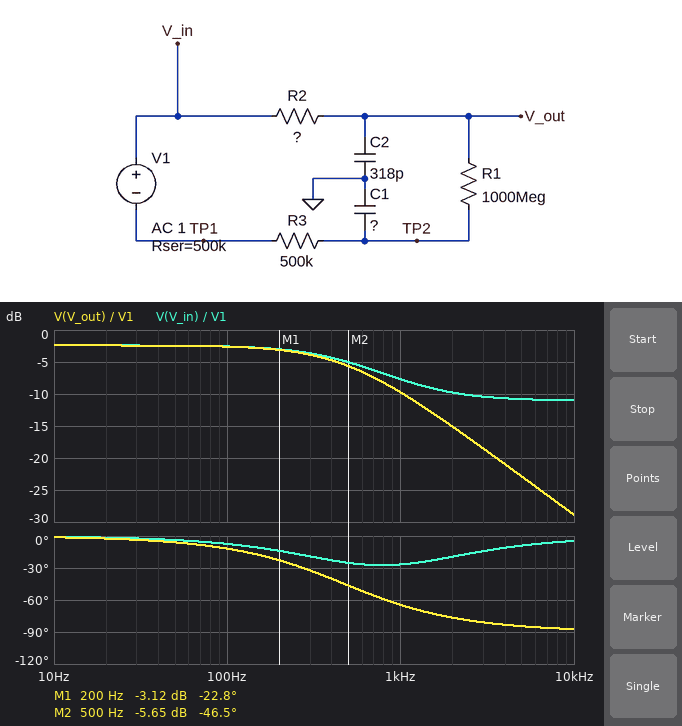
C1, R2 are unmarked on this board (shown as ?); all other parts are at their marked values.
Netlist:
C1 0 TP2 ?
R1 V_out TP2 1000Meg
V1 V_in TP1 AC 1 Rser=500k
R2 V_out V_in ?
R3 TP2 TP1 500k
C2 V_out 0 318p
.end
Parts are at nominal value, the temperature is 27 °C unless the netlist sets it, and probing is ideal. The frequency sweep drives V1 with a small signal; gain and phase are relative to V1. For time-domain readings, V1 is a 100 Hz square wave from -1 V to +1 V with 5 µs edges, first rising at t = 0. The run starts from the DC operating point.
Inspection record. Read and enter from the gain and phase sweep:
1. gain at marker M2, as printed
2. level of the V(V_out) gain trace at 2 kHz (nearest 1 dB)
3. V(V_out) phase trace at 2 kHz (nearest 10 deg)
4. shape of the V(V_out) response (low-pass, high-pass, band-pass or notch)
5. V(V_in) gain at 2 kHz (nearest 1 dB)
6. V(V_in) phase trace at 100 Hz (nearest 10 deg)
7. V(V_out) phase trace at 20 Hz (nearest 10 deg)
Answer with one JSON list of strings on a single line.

["-5.65 dB", "-15 dB", "-80 deg", "low-pass", "-10 dB", "-10 deg", "0 deg"]
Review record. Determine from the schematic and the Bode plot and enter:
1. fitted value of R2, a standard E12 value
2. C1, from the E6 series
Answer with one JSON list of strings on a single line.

["390 kΩ", "1 nF"]
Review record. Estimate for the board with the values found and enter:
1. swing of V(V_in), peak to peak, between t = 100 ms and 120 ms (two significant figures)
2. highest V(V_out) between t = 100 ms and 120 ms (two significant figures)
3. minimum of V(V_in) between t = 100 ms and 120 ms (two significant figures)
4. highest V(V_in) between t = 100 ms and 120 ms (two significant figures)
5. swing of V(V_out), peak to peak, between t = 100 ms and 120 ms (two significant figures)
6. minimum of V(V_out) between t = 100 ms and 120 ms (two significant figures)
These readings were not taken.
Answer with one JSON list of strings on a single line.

["1.5 V", "1.6 V", "57 mV", "1.6 V", "1.5 V", "57 mV"]
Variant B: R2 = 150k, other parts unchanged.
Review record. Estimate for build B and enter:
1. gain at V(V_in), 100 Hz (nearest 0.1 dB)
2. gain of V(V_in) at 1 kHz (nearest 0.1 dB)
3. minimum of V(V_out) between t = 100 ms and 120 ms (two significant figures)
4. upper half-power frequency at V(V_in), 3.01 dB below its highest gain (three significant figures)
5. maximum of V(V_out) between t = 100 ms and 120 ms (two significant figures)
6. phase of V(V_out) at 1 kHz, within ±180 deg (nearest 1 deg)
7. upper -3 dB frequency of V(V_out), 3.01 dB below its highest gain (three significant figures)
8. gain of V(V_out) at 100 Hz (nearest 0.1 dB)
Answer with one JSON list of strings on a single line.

["-2.5 dB", "-8.1 dB", "24 mV", "592 Hz", "1.5 V", "-60 deg", "574 Hz", "-2.5 dB"]
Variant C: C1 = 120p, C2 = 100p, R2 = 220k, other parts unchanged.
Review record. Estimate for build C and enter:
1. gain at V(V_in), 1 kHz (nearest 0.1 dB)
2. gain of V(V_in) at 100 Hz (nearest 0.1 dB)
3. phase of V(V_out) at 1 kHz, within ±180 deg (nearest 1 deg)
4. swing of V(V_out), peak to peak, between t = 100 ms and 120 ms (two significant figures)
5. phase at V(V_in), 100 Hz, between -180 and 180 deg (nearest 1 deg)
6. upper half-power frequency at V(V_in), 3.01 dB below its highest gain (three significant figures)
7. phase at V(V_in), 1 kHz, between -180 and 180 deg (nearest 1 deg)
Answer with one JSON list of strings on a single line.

["-5.9 dB", "-5.3 dB", "-23 deg", "1.1 V", "-2 deg", "2.71 kHz", "-15 deg"]
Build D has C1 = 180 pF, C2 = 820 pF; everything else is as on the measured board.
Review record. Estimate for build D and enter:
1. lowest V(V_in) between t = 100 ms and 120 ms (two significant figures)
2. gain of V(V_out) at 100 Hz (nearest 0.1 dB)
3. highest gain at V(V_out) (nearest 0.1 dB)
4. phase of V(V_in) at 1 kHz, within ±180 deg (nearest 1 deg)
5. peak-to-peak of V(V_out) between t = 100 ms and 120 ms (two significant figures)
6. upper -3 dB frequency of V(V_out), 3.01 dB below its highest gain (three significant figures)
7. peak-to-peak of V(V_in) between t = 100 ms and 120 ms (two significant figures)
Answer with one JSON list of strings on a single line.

["-140 mV", "-15.0 dB", "-14.9 dB", "11 deg", "360 mV", "777 Hz", "760 mV"]
